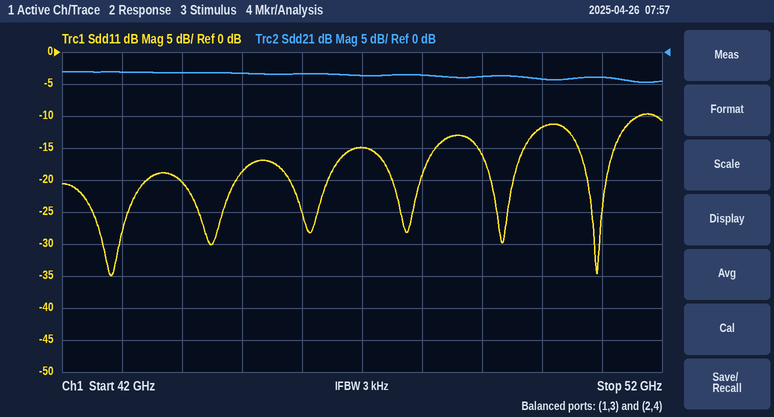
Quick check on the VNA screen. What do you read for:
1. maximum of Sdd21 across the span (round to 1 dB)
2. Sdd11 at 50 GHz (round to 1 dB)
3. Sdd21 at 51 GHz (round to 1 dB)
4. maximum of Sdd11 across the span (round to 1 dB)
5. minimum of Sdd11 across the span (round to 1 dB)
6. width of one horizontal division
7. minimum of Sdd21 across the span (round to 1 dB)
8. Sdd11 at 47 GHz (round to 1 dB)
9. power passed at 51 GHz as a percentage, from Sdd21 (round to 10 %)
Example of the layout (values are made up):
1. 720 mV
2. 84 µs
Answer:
1. -3 dB
2. -12 dB
3. -4 dB
4. -10 dB
5. -35 dB
6. 1 GHz
7. -5 dB
8. -15 dB
9. 40 %
